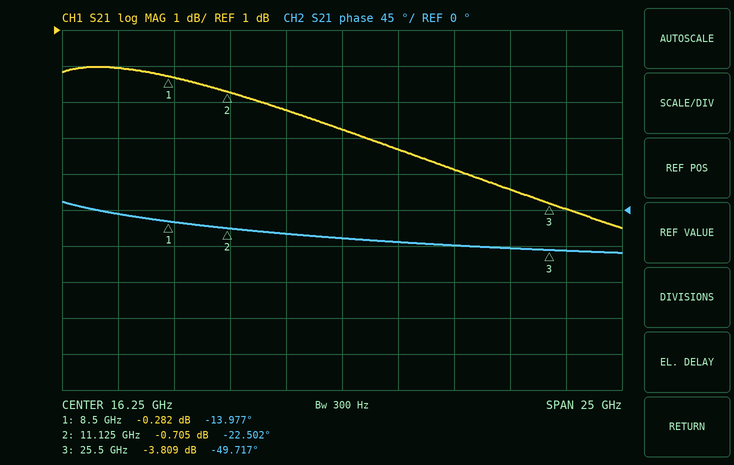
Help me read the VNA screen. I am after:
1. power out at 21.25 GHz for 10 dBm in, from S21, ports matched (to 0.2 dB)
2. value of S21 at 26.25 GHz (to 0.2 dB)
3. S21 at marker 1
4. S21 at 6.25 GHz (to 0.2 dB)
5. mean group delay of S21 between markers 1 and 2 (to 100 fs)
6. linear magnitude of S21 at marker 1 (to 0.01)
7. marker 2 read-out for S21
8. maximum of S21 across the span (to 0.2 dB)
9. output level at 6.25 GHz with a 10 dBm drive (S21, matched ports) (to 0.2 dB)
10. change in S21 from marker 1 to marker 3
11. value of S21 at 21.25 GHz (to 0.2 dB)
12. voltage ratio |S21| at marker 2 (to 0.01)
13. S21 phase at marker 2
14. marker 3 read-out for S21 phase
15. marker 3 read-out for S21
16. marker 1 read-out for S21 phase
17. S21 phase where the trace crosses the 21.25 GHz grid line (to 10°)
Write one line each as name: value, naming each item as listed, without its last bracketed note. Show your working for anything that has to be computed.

power out at 21.25 GHz for 10 dBm in, from S21, ports matched: 10 dBm + (-2.8 dB) = 7.2 dBm
value of S21 at 26.25 GHz: -4.0 dB
S21 at marker 1: -0.282 dB
S21 at 6.25 GHz: 0.0 dB
mean group delay of S21 between markers 1 and 2: −(-22.502° − (-13.977°))/(360° × 2.625 GHz) ≈ 9.0 ps
linear magnitude of S21 at marker 1: 10^(-0.282/20) ≈ 0.97
marker 2 read-out for S21: -0.705 dB
maximum of S21 across the span: 0.0 dB
output level at 6.25 GHz with a 10 dBm drive (S21, matched ports): 10 dBm + (0.0 dB) = 10.0 dBm
change in S21 from marker 1 to marker 3: -3.809 − (-0.282) = -3.527 dB
value of S21 at 21.25 GHz: -2.8 dB
voltage ratio |S21| at marker 2: 10^(-0.705/20) ≈ 0.92
S21 phase at marker 2: -22.502°
marker 3 read-out for S21 phase: -49.717°
marker 3 read-out for S21: -3.809 dB
marker 1 read-out for S21 phase: -13.977°
S21 phase where the trace crosses the 21.25 GHz grid line: -40°
